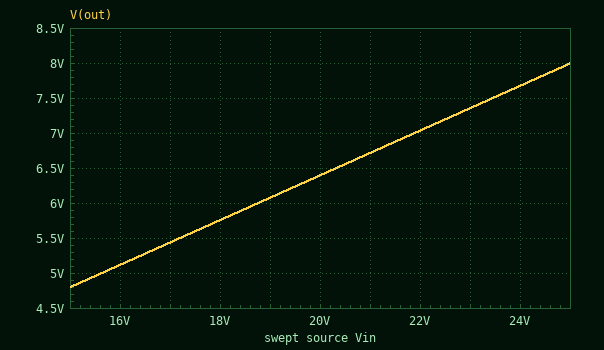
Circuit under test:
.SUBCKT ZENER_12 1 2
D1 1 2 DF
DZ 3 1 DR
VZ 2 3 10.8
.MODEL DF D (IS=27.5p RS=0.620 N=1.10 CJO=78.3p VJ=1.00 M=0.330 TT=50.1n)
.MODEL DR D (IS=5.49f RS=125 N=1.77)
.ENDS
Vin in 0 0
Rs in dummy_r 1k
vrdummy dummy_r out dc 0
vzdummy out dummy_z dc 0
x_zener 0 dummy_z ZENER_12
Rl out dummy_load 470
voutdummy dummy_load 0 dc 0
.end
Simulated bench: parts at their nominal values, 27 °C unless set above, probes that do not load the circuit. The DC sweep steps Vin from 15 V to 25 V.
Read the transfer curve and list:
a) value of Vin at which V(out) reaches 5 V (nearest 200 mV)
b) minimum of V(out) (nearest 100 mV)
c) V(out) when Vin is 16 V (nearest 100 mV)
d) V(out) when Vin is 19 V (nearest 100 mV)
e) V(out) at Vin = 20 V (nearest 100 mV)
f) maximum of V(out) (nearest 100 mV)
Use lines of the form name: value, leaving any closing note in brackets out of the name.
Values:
value of Vin at which V(out) reaches 5 V: 15.6 V
minimum of V(out): 4.8 V
V(out) when Vin is 16 V: 5.1 V
V(out) when Vin is 19 V: 6.1 V
V(out) at Vin = 20 V: 6.4 V
maximum of V(out): 8.0 V
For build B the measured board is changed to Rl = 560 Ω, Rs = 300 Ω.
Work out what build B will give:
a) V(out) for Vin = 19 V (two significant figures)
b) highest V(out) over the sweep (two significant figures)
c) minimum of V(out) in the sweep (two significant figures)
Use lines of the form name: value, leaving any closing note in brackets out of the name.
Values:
V(out) for Vin = 19 V: 12 V
highest V(out) over the sweep: 14 V
minimum of V(out) in the sweep: 9.8 V
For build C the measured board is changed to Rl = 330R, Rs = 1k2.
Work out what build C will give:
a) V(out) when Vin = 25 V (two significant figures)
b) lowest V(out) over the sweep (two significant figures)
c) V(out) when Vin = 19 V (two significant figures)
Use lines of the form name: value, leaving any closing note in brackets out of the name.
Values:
V(out) when Vin = 25 V: 5.4 V
lowest V(out) over the sweep: 3.2 V
V(out) when Vin = 19 V: 4.1 V
